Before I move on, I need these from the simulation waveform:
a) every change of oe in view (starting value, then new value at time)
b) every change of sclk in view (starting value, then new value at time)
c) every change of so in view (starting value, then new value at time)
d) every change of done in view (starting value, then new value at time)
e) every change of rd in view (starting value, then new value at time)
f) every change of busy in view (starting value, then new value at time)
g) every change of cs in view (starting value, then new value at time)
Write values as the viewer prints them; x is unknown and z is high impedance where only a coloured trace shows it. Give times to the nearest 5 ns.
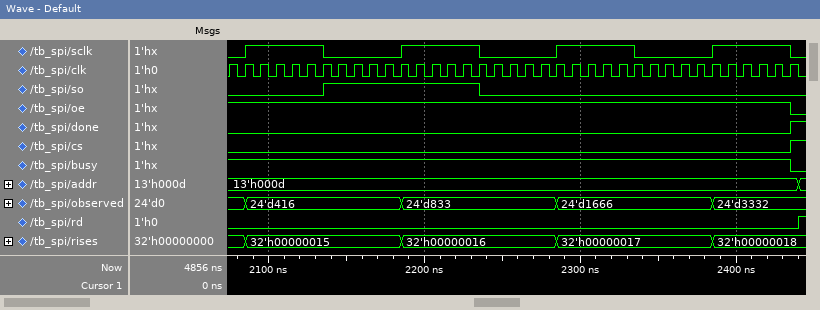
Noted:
1, 0 at 2435 ns
0, 1 at 2085 ns, 0 at 2135 ns, 1 at 2185 ns, 0 at 2235 ns, 1 at 2285 ns, 0 at 2335 ns, 1 at 2385 ns, 0 at 2435 ns
0, 1 at 2135 ns, 0 at 2235 ns
0, 1 at 2435 ns
0, 1 at 2440 ns
1, 0 at 2435 ns
0, 1 at 2435 ns
